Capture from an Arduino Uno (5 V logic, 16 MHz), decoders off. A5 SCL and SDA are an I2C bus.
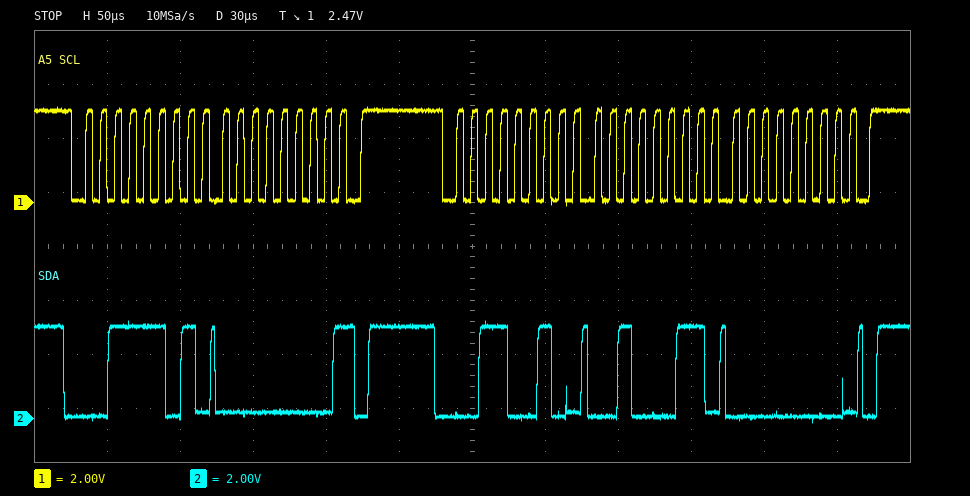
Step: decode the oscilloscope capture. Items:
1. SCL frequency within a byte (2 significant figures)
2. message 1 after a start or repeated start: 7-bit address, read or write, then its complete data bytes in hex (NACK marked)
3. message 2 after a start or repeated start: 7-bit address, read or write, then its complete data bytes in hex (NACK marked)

100 kHz
0x1E read: 00 NACK
0x19 write: 23 00
